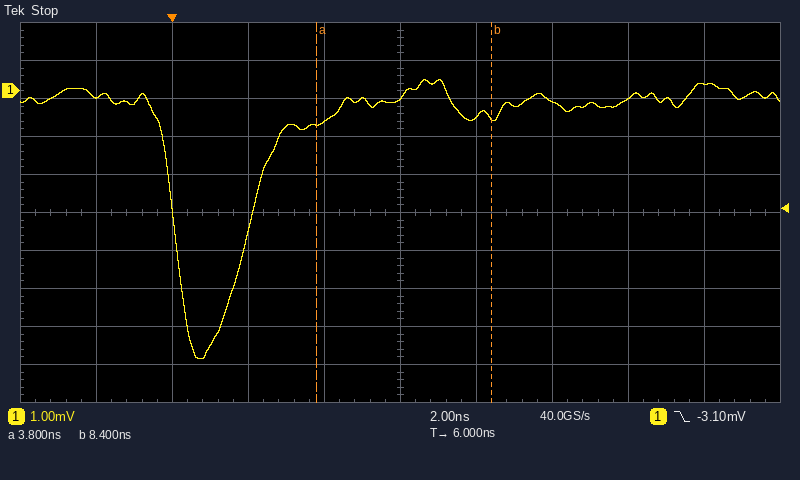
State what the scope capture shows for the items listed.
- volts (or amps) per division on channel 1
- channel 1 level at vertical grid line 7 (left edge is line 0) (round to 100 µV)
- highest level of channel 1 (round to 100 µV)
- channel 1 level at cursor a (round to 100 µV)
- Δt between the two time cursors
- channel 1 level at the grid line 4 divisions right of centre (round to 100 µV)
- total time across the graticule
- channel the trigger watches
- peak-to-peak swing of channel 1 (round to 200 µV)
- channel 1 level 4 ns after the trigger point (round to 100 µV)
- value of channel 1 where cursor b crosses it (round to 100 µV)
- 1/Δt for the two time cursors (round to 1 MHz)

1 mV
-300 µV
300 µV
-900 µV
4.6 ns
200 µV
20 ns
channel 1
7.4 mV
-800 µV
-700 µV
217 MHz
